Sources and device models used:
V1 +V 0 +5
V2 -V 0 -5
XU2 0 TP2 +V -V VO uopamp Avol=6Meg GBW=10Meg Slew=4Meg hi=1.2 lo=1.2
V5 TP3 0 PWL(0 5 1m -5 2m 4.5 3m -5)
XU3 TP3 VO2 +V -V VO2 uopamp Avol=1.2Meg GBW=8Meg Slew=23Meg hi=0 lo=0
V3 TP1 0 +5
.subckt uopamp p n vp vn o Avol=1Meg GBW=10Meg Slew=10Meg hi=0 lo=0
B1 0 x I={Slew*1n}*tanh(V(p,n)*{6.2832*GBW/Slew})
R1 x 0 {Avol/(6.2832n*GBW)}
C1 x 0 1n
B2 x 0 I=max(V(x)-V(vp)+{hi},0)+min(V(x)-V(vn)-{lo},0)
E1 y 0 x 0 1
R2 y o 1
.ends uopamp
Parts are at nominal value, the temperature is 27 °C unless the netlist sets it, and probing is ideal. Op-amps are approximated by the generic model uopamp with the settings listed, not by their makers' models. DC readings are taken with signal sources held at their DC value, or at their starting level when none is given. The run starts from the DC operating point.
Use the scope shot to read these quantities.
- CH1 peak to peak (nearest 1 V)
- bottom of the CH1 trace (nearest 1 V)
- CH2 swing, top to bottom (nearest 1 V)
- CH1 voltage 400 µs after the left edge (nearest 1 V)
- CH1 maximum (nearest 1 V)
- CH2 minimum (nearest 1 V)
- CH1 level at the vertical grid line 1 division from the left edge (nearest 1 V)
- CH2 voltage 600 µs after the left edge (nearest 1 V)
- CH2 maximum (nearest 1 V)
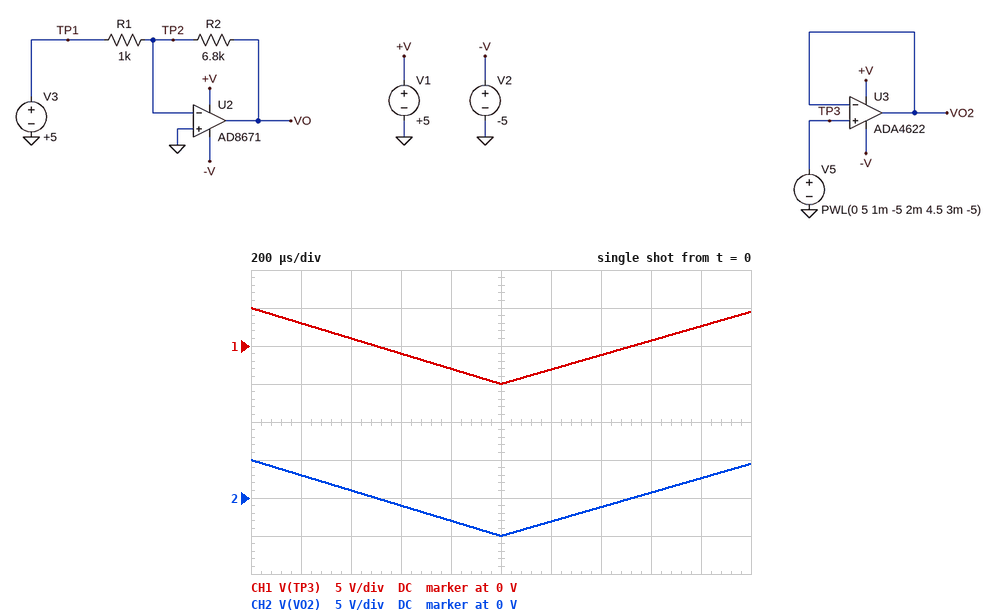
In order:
10 V
-5 V
10 V
1 V
5 V
-5 V
3 V
-1 V
5 V
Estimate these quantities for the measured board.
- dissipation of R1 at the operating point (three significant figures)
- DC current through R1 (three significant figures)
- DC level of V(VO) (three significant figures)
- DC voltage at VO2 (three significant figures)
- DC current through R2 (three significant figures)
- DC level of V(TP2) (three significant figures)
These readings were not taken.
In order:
1.27 mW
1.13 mA
-3.80 V
5.00 V
1.13 mA
3.87 V
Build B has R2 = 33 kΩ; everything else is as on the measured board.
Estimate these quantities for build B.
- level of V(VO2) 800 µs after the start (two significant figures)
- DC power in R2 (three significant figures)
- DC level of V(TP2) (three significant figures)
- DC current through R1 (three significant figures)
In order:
-3.0 V
2.21 mW
4.74 V
259 µA
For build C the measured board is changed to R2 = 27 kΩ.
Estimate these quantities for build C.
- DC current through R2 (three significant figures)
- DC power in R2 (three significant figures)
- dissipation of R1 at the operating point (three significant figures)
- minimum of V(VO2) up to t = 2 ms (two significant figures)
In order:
314 µA
2.67 mW
98.9 µW
-5.0 V
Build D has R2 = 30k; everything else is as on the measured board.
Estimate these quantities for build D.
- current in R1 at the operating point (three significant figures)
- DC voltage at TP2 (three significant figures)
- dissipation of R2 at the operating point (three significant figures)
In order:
284 µA
4.72 V
2.42 mW
